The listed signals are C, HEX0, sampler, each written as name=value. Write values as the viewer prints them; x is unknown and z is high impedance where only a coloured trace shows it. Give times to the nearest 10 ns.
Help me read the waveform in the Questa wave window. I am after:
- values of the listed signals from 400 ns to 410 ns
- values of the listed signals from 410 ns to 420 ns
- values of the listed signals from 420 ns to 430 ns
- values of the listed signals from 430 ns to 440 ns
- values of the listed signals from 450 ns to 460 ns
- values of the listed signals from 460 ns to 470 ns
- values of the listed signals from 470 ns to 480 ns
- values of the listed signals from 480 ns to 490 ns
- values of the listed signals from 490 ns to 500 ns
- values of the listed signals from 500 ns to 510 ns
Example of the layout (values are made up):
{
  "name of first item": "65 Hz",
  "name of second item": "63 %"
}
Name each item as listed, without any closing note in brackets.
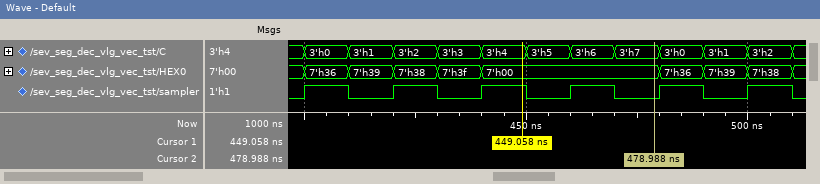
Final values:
{
  "values of the listed signals from 400 ns to 410 ns": "C=3'h0, HEX0=7'h36, sampler=1",
  "values of the listed signals from 410 ns to 420 ns": "C=3'h1, HEX0=7'h39, sampler=0",
  "values of the listed signals from 420 ns to 430 ns": "C=3'h2, HEX0=7'h38, sampler=1",
  "values of the listed signals from 430 ns to 440 ns": "C=3'h3, HEX0=7'h3f, sampler=0",
  "values of the listed signals from 450 ns to 460 ns": "C=3'h5, HEX0=7'h00, sampler=0",
  "values of the listed signals from 460 ns to 470 ns": "C=3'h6, HEX0=7'h00, sampler=1",
  "values of the listed signals from 470 ns to 480 ns": "C=3'h7, HEX0=7'h00, sampler=0",
  "values of the listed signals from 480 ns to 490 ns": "C=3'h0, HEX0=7'h36, sampler=1",
  "values of the listed signals from 490 ns to 500 ns": "C=3'h1, HEX0=7'h39, sampler=0",
  "values of the listed signals from 500 ns to 510 ns": "C=3'h2, HEX0=7'h38, sampler=1"
}
